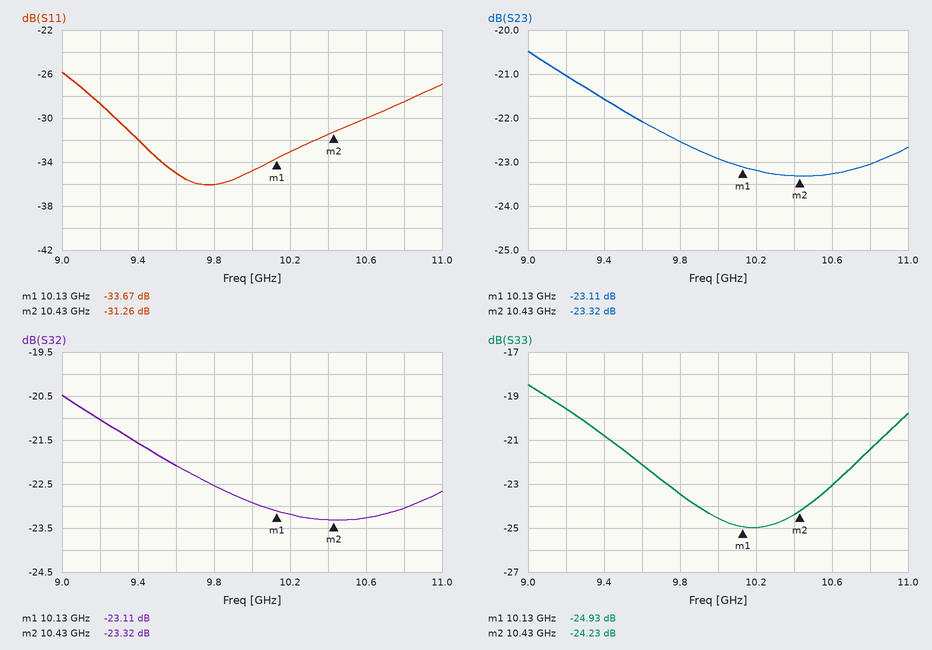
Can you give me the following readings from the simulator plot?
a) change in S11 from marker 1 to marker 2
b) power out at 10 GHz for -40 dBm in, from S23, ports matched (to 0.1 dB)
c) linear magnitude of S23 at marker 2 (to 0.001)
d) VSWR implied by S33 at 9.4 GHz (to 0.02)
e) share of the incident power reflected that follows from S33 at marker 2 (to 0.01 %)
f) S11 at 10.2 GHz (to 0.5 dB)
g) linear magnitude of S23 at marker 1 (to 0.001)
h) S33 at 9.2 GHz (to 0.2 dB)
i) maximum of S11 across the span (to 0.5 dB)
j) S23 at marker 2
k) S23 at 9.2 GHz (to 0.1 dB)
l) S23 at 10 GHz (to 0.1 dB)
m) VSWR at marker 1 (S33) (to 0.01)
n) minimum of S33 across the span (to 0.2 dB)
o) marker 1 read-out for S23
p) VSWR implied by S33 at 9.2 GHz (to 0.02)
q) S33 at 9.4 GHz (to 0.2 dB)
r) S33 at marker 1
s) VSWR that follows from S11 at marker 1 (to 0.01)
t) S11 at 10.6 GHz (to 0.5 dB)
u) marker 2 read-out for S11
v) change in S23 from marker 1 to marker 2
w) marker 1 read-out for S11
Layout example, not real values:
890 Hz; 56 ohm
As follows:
2.41 dB; -62.9 dBm; 0.068; 1.20; 0.38 %; -33.0 dB; 0.070; -19.6 dB; -26.0 dB; -23.32 dB; -21.0 dB; -22.9 dB; 1.12; -25.0 dB; -23.11 dB; 1.24; -20.8 dB; -24.93 dB; 1.04; -30.0 dB; -31.26 dB; -0.21 dB; -33.67 dB
